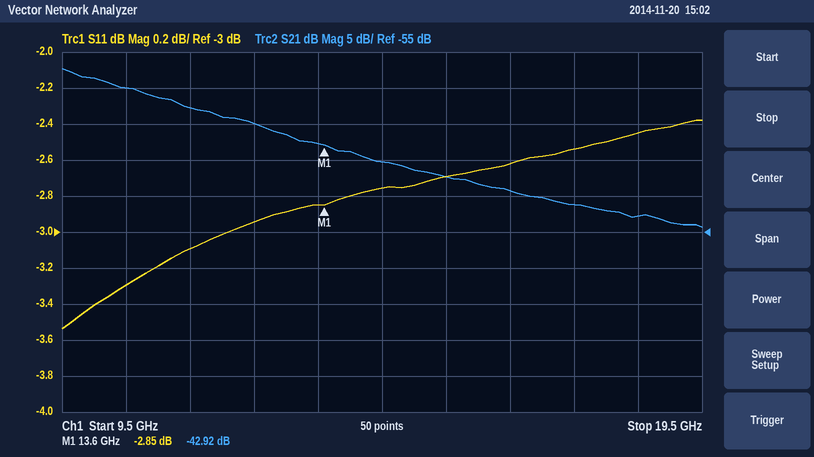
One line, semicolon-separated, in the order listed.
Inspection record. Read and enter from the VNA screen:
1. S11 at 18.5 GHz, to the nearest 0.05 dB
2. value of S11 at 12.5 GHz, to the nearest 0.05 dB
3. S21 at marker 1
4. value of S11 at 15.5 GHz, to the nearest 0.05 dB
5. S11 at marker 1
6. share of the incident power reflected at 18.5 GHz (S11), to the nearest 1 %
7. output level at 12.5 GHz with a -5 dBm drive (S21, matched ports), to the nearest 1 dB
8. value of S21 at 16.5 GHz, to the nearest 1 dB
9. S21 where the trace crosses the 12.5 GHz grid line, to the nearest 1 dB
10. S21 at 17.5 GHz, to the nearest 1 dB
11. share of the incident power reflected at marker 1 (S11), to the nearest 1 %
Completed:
-2.45 dB; -2.95 dB; -42.92 dB; -2.70 dB; -2.85 dB; 57 %; -45 dBm; -49 dB; -40 dB; -51 dB; 52 %
